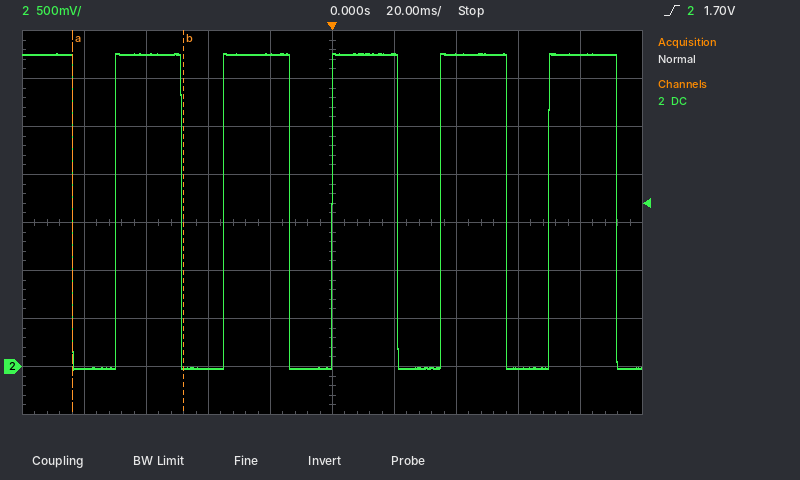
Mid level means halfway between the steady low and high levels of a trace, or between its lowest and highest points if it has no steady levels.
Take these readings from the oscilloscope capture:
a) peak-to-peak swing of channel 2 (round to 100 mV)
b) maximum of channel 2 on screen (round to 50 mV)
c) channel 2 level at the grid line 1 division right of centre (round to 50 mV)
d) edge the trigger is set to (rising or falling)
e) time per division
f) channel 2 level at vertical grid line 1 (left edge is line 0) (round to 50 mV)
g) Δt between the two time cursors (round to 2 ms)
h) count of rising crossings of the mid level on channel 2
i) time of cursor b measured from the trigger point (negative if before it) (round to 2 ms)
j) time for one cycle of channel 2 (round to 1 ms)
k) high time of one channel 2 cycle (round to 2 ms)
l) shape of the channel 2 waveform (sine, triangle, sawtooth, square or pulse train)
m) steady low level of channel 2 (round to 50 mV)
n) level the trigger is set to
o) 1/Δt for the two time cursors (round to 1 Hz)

3.30 V
3.25 V
3.25 V
rising
20 ms
0 mV
36 ms
5
-48 ms
35 ms
22 ms
pulse train
0 mV
1.70 V
28 Hz
